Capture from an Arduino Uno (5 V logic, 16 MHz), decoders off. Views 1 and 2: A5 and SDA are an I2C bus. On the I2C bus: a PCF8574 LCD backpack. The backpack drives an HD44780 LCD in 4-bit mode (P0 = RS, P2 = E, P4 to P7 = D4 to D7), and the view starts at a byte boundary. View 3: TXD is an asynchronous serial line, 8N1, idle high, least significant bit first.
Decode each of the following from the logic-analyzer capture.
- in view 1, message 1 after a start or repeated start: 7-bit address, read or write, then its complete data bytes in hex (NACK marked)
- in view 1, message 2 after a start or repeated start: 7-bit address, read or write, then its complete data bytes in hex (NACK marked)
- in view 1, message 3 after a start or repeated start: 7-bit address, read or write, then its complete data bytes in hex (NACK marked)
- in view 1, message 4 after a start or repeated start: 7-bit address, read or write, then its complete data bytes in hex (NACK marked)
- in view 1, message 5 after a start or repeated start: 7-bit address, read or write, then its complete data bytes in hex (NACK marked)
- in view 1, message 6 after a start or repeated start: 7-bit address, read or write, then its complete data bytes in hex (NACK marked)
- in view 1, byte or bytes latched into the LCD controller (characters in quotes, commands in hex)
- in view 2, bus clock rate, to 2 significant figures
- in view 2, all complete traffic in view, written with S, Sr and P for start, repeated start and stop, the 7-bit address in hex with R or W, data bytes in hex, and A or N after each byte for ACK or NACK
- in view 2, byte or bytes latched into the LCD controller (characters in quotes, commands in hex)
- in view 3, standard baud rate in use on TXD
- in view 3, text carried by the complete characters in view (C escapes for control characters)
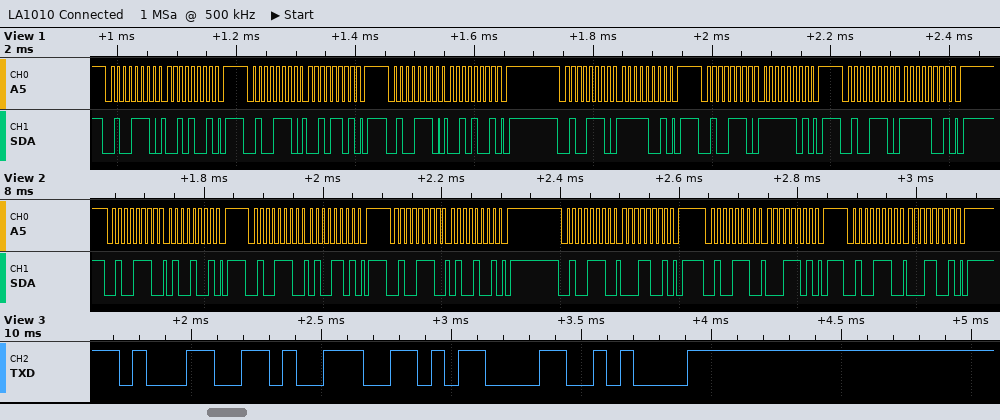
0x27 write: 29
0x27 write: 2D
0x27 write: 29
0x27 write: F9
0x27 write: FD
0x27 write: F9
'/'
100 kHz
S 27W A 49 A P S 27W A 4D A P S 27W A 49 A P S 27W A 19 A P S 27W A 1D A P S 27W A 19 A P
'A'
19200 baud
"19\r\n"
